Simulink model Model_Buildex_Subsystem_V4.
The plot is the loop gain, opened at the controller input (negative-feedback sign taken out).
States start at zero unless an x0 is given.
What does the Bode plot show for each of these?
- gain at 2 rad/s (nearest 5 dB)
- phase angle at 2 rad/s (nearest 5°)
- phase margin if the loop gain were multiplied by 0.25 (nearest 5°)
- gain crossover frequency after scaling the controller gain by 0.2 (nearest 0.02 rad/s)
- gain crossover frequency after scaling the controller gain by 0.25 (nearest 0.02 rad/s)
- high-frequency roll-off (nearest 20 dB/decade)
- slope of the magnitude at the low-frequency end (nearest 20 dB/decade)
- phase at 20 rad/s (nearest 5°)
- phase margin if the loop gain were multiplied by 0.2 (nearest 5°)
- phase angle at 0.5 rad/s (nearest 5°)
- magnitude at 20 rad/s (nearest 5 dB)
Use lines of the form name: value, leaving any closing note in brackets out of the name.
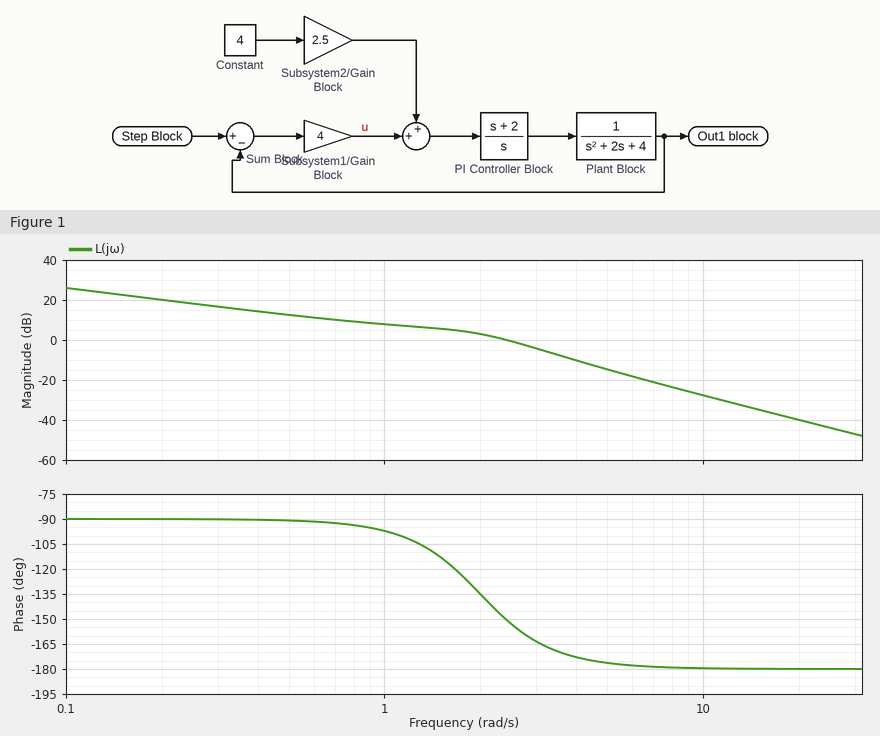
gain at 2 rad/s: 5 dB
phase angle at 2 rad/s: -135°
phase margin if the loop gain were multiplied by 0.25: 90°
gain crossover frequency after scaling the controller gain by 0.2: 0.42 rad/s
gain crossover frequency after scaling the controller gain by 0.25: 0.54 rad/s
high-frequency roll-off: -40 dB/decade
slope of the magnitude at the low-frequency end: -20 dB/decade
phase at 20 rad/s: -180°
phase margin if the loop gain were multiplied by 0.2: 90°
phase angle at 0.5 rad/s: -90°
magnitude at 20 rad/s: -40 dB
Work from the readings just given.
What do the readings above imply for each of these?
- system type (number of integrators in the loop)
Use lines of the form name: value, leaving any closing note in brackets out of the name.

system type: 1
